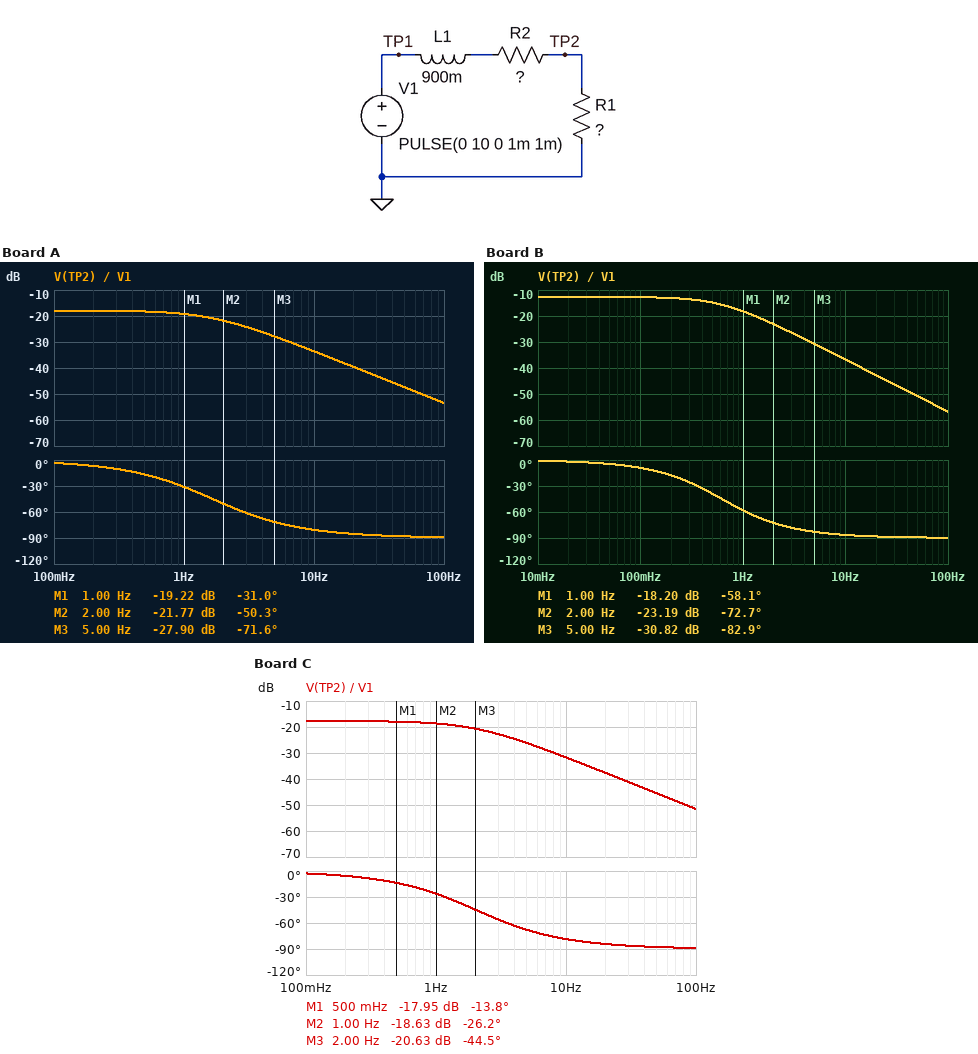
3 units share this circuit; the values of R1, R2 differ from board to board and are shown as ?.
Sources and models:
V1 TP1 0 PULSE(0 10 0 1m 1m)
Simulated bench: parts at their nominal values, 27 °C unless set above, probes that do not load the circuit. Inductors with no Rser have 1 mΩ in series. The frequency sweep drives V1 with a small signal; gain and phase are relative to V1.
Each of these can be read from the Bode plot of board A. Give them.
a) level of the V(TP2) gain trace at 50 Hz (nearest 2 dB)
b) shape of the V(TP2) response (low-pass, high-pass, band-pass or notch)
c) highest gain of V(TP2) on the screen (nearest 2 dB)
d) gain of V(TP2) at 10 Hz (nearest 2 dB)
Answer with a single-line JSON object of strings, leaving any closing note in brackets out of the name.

{"level of the V(TP2) gain trace at 50 Hz": "-48 dB", "shape of the V(TP2) response": "low-pass", "highest gain of V(TP2) on the screen": "-18 dB", "gain of V(TP2) at 10 Hz": "-34 dB"}
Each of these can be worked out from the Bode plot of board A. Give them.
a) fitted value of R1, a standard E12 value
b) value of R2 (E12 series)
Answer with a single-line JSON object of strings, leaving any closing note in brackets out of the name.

{"fitted value of R1, a standard E12 value": "1.2 Ω", "value of R2": "8.2 Ω"}
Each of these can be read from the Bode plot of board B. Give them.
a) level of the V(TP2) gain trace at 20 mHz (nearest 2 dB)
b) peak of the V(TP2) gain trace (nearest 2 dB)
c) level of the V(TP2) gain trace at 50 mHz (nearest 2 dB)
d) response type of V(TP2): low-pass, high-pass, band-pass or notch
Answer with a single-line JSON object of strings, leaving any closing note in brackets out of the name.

{"level of the V(TP2) gain trace at 20 mHz": "-12 dB", "peak of the V(TP2) gain trace": "-12 dB", "level of the V(TP2) gain trace at 50 mHz": "-12 dB", "response type of V(TP2): low-pass, high-pass, band-pass or notch": "low-pass"}
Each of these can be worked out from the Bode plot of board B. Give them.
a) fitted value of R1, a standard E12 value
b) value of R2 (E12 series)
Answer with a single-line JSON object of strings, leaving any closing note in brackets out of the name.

{"fitted value of R1, a standard E12 value": "0.82 Ω", "value of R2": "2.7 Ω"}
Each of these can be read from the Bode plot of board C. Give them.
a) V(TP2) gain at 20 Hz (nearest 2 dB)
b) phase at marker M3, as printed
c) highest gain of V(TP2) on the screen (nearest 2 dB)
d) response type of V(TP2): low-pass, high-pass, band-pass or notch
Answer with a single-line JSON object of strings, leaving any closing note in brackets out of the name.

{"V(TP2) gain at 20 Hz": "-38 dB", "phase at marker M3, as printed": "-44.5 deg", "highest gain of V(TP2) on the screen": "-18 dB", "response type of V(TP2): low-pass, high-pass, band-pass or notch": "low-pass"}
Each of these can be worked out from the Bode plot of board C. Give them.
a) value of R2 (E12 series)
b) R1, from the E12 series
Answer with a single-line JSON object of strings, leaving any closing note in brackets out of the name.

{"value of R2": "10 Ω", "R1, from the E12 series": "1.5 Ω"}
